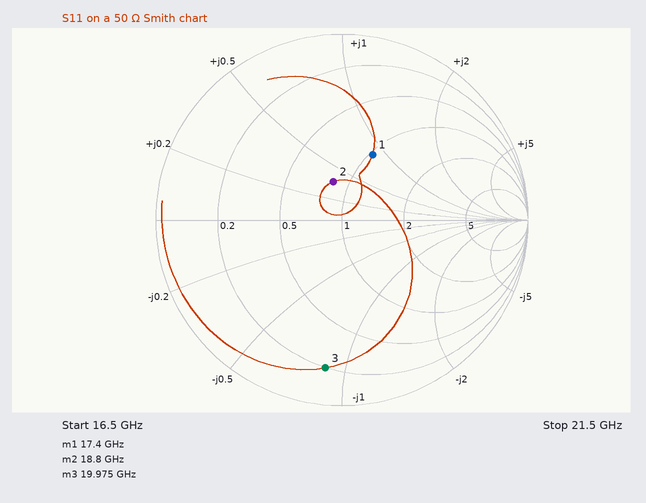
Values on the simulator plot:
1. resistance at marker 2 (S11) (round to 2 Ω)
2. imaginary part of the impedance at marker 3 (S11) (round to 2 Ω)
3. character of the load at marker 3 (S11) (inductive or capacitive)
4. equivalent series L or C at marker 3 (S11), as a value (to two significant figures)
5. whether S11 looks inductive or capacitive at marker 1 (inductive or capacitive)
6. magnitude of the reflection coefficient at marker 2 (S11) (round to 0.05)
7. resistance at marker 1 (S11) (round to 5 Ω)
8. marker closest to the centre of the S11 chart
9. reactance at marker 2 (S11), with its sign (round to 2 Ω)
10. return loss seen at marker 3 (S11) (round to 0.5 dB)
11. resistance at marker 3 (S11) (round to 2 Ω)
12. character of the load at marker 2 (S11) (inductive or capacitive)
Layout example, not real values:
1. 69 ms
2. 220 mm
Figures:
1. 42 Ω
2. -44 Ω
3. capacitive
4. 180 fF
5. inductive
6. 0.20
7. 50 Ω
8. marker 2
9. +18 Ω
10. 2.0 dB
11. 10 Ω
12. inductive
